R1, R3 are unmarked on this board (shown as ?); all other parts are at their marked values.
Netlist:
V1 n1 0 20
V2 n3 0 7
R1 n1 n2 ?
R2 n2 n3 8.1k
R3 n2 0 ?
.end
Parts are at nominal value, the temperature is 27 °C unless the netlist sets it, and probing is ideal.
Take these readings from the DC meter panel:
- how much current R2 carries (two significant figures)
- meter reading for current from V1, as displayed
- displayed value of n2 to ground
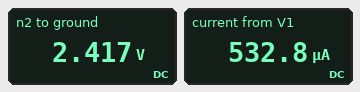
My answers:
570 µA
532.8 µA
2.417 V
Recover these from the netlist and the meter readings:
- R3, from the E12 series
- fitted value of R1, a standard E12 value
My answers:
2.2 kΩ
33 kΩ
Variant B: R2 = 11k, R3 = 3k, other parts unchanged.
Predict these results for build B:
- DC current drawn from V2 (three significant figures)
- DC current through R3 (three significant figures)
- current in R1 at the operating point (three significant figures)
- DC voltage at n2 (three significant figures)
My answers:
388 µA
911 µA
523 µA
2.73 V
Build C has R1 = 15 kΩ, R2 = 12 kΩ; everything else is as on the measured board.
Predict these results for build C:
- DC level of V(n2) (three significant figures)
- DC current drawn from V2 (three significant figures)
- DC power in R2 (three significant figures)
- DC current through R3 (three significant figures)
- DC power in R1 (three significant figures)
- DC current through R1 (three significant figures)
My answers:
3.17 V
319 µA
1.22 mW
1.44 mA
18.9 mW
1.12 mA
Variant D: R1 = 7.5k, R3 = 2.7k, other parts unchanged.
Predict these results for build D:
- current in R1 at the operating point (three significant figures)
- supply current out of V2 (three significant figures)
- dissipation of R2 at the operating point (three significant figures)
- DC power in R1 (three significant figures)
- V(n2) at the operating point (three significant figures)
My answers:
1.92 mA
169 µA
232 µW
27.5 mW
5.63 V
